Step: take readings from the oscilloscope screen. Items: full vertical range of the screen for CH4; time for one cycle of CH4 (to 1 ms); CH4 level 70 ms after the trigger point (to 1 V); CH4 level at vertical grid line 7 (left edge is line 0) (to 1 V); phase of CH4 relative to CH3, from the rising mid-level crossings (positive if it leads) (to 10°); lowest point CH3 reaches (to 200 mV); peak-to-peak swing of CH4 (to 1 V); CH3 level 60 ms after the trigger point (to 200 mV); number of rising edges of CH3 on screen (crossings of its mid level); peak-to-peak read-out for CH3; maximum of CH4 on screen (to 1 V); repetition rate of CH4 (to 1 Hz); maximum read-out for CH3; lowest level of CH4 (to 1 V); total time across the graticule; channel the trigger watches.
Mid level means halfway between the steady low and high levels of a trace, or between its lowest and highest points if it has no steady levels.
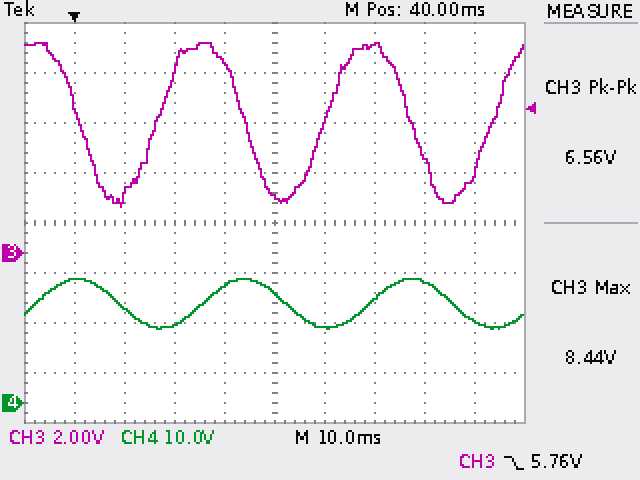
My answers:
80 V
33 ms
24 V
21 V
-100°
1.8 V
10 V
8.4 V
3
6.56 V
25 V
30 Hz
8.44 V
15 V
100 ms
CH3
